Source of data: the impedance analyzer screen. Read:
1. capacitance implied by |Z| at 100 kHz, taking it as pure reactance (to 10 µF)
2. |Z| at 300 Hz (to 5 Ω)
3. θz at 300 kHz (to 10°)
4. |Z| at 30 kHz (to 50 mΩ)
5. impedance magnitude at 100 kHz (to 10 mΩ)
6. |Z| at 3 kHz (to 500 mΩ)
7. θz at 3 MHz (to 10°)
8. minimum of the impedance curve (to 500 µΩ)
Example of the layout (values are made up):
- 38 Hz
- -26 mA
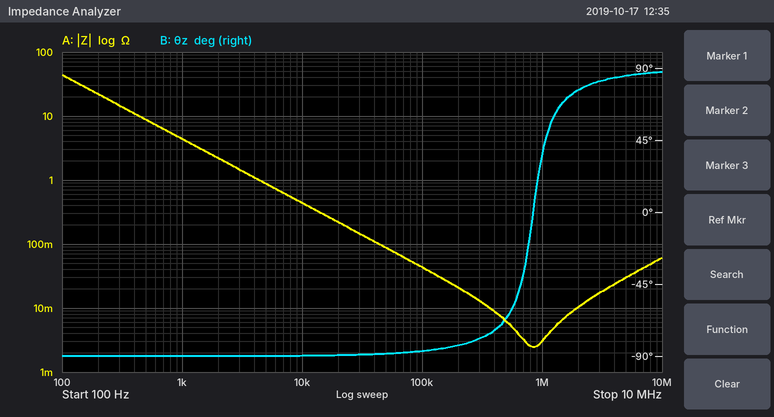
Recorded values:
- 40 µF
- 15 Ω
- -80°
- 150 mΩ
- 40 mΩ
- 1.5 Ω
- 80°
- 2.5 mΩ
